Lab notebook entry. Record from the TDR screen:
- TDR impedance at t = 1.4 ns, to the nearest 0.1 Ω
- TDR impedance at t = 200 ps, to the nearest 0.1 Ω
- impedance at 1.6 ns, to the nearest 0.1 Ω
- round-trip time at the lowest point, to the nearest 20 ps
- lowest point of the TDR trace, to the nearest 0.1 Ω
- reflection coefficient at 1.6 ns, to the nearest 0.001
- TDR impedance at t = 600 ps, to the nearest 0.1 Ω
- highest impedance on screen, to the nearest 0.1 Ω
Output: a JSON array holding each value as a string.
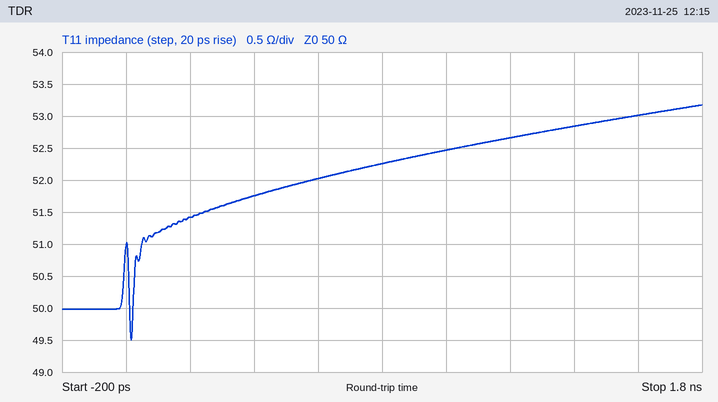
["52.8 Ω", "51.4 Ω", "53.0 Ω", "20 ps", "49.5 Ω", "+0.029", "52.0 Ω", "53.2 Ω"]
